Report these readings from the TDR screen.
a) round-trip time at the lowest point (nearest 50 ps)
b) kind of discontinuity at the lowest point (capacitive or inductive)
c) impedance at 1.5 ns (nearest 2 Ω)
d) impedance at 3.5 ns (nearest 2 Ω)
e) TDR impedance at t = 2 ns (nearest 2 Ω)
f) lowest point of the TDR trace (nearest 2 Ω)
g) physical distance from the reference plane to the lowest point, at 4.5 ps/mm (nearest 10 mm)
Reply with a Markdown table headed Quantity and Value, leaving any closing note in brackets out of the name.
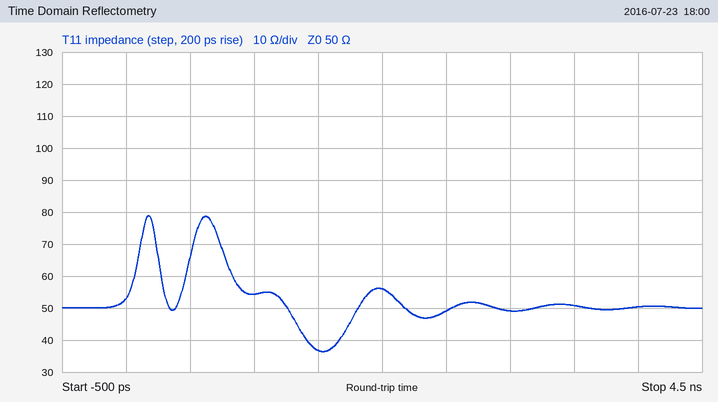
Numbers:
| Quantity | Value |
|---|---|
| round-trip time at the lowest point | 1.55 ns |
| kind of discontinuity at the lowest point | capacitive |
| impedance at 1.5 ns | 36 Ω |
| impedance at 3.5 ns | 50 Ω |
| TDR impedance at t = 2 ns | 56 Ω |
| lowest point of the TDR trace | 36 Ω |
| physical distance from the reference plane to the lowest point, at 4.5 ps/mm | 170 mm |
